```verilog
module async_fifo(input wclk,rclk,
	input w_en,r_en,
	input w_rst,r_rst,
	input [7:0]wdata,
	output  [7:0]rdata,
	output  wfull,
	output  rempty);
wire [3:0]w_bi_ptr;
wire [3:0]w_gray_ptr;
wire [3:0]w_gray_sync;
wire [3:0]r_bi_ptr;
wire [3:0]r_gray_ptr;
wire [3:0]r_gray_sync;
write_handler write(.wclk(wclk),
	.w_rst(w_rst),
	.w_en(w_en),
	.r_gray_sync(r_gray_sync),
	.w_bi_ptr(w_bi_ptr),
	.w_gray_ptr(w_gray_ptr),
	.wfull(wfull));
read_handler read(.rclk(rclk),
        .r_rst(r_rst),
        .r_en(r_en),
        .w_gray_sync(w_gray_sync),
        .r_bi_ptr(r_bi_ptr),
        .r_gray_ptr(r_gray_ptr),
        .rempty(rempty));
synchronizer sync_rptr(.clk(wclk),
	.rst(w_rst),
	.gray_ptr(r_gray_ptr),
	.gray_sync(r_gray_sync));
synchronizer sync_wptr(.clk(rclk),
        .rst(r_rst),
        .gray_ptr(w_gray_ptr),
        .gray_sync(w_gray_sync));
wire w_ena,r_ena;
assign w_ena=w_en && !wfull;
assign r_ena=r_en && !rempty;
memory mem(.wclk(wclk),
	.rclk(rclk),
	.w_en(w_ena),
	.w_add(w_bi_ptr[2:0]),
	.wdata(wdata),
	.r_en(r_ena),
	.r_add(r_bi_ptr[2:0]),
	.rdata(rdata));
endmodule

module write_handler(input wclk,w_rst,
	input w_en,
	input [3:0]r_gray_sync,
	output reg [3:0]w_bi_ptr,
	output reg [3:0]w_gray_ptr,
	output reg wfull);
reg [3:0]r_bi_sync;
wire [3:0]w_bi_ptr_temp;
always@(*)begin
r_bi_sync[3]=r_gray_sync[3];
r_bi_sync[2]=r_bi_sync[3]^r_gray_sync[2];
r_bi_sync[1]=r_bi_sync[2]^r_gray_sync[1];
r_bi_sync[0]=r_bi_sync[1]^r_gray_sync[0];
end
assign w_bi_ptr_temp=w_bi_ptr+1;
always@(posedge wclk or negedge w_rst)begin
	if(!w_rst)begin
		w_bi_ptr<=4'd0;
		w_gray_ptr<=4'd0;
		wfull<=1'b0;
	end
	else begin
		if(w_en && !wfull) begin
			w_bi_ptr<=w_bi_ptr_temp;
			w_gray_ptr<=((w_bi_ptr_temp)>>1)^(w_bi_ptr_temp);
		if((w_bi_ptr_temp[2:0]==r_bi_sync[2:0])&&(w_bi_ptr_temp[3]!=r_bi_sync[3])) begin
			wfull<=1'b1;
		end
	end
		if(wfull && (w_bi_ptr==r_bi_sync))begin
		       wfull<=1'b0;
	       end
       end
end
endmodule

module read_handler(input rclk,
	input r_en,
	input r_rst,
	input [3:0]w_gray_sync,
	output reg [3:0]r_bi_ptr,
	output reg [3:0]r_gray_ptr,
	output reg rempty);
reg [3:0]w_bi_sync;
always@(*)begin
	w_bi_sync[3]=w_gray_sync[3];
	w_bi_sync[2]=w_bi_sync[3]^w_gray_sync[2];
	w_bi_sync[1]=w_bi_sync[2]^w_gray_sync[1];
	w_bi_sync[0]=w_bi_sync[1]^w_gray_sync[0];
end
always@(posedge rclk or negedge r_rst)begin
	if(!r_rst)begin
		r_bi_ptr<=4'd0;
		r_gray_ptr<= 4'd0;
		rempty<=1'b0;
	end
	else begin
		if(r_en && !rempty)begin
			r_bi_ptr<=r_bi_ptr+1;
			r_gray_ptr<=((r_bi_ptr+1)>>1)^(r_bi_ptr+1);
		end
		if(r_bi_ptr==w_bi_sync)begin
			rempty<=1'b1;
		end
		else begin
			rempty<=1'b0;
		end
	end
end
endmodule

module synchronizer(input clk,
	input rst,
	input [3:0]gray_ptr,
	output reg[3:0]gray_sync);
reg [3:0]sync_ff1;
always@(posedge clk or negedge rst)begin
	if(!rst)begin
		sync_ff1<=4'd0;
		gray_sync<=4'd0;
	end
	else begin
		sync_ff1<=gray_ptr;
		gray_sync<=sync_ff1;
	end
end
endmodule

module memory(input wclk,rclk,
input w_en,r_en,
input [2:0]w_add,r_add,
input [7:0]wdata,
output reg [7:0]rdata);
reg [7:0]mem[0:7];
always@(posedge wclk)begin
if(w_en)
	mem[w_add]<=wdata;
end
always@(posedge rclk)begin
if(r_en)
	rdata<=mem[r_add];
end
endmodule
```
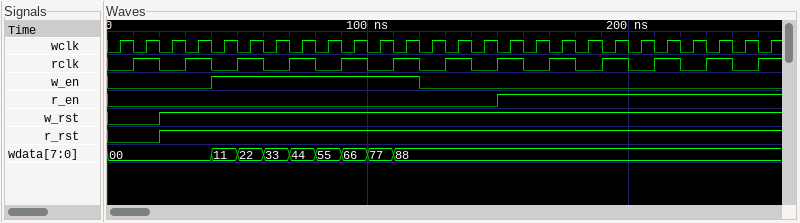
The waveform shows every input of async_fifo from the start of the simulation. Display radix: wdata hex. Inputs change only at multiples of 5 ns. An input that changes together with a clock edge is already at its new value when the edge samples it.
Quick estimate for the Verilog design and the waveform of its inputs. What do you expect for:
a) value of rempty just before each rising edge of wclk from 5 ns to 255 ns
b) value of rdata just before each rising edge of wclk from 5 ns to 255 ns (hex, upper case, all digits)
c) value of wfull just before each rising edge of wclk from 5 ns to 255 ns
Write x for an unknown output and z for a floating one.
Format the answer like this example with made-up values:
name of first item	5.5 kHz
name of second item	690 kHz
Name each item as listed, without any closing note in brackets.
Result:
value of rempty just before each rising edge of wclk from 5 ns to 255 ns	0 0 0 1 1 1 1 1 1 0 0 0 0 0 0 0 0 0 0 0 0 0 0 0 0 0
value of rdata just before each rising edge of wclk from 5 ns to 255 ns	x, x, x, x, x, x, x, x, x, x, x, x, x, x, x, 11, 11, 22, 22, 33, 33, 44, 44, 55, 55, 66
value of wfull just before each rising edge of wclk from 5 ns to 255 ns	0 0 0 0 0 0 0 0 0 0 0 0 1 1 1 1 1 1 1 1 1 1 1 1 1 1
